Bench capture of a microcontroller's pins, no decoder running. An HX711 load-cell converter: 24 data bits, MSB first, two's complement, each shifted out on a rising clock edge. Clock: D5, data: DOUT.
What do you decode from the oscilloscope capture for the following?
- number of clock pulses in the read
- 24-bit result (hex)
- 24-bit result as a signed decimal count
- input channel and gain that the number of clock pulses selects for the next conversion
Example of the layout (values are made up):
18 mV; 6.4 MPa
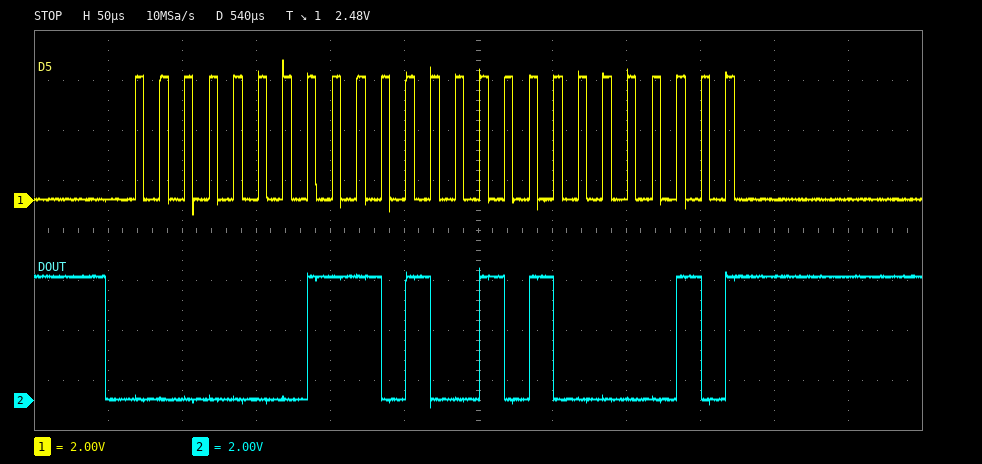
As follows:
25; 0x01D282; 119426; channel A, gain 128
